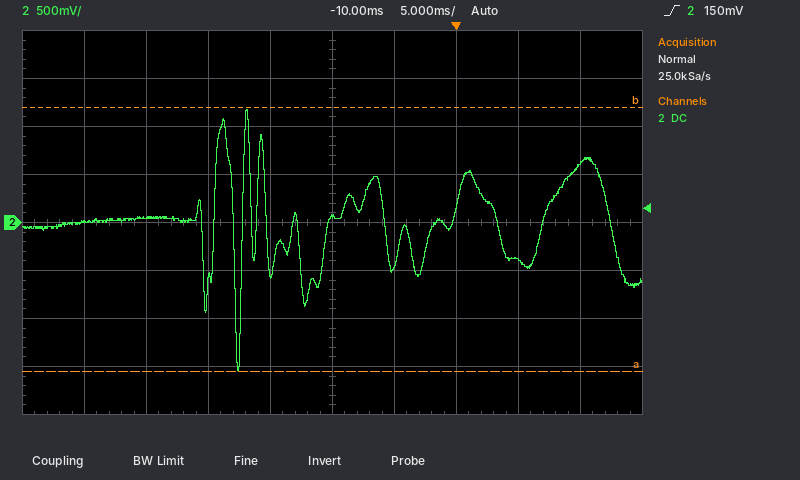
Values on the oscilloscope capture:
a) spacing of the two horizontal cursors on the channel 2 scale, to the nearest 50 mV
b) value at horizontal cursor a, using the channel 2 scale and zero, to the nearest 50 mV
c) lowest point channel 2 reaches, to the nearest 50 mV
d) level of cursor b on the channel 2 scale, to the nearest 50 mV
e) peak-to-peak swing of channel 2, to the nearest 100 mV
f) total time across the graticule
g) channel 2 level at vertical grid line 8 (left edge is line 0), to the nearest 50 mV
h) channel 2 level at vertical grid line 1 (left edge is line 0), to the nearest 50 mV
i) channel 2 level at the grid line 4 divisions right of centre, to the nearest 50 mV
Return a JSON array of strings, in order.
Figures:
["2.75 V", "-1.55 V", "-1.55 V", "1.20 V", "2.70 V", "50 ms", "-400 mV", "0 mV", "600 mV"]
